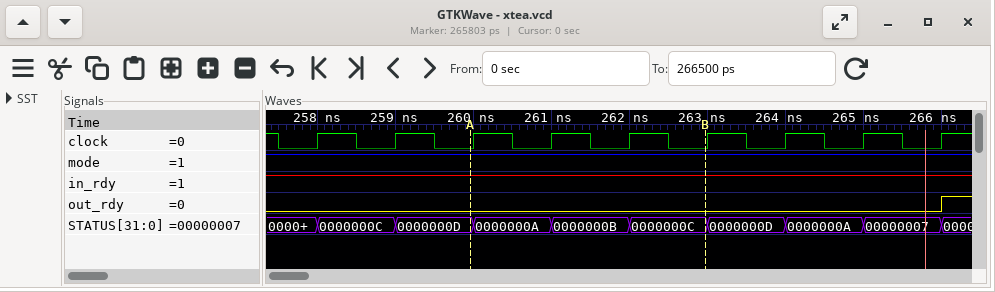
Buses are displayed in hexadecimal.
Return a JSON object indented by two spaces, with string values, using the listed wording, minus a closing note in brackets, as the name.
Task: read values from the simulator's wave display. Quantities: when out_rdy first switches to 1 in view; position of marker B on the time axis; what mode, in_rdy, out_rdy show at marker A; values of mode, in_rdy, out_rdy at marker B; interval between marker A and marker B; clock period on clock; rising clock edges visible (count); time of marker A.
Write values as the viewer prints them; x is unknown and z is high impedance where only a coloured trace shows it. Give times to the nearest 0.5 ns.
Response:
{
  "when out_rdy first switches to 1 in view": "266 ns",
  "position of marker B on the time axis": "263 ns",
  "what mode, in_rdy, out_rdy show at marker A": "mode=1, in_rdy=1, out_rdy=0",
  "values of mode, in_rdy, out_rdy at marker B": "mode=1, in_rdy=1, out_rdy=0",
  "interval between marker A and marker B": "3 ns",
  "clock period on clock": "1 ns",
  "rising clock edges visible": "9",
  "time of marker A": "260 ns"
}
